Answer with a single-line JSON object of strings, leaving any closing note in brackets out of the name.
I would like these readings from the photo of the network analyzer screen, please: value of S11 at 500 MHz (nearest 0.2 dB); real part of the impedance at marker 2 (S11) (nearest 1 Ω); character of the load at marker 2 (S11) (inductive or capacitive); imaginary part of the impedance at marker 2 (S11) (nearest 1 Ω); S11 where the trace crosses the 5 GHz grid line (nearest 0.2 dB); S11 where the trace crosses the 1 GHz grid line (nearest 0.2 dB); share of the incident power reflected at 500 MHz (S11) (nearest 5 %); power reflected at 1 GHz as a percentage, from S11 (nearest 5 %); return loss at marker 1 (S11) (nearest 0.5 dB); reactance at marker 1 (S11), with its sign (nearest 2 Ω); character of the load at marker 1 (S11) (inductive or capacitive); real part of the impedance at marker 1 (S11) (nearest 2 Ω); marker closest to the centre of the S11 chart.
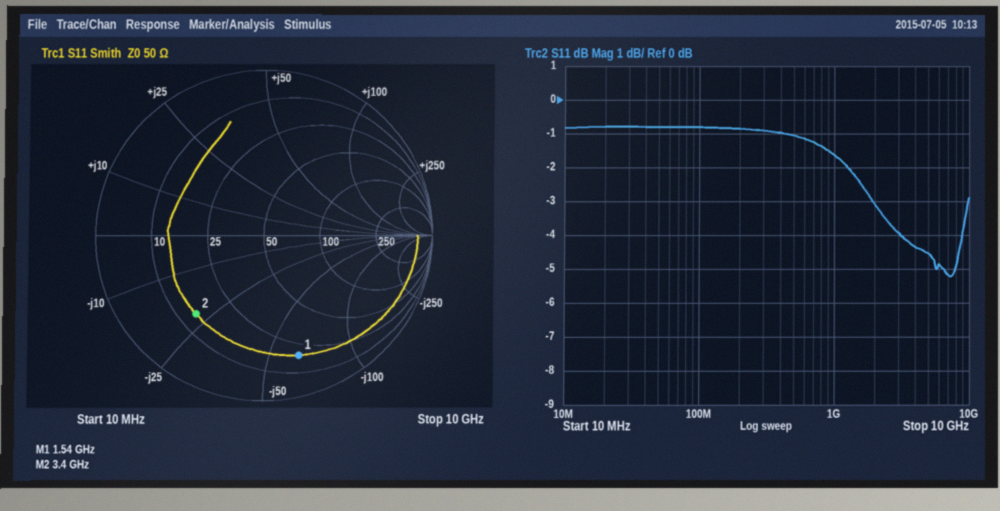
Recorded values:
{"value of S11 at 500 MHz": "-1.0 dB", "real part of the impedance at marker 2 (S11)": "14 Ω", "character of the load at marker 2 (S11)": "capacitive", "imaginary part of the impedance at marker 2 (S11)": "-22 Ω", "S11 where the trace crosses the 5 GHz grid line": "-4.6 dB", "S11 where the trace crosses the 1 GHz grid line": "-1.6 dB", "share of the incident power reflected at 500 MHz (S11)": "80 %", "power reflected at 1 GHz as a percentage, from S11": "70 %", "return loss at marker 1 (S11)": "2.5 dB", "reactance at marker 1 (S11), with its sign": "-64 Ω", "character of the load at marker 1 (S11)": "capacitive", "real part of the impedance at marker 1 (S11)": "18 Ω", "marker closest to the centre of the S11 chart": "marker 2"}
